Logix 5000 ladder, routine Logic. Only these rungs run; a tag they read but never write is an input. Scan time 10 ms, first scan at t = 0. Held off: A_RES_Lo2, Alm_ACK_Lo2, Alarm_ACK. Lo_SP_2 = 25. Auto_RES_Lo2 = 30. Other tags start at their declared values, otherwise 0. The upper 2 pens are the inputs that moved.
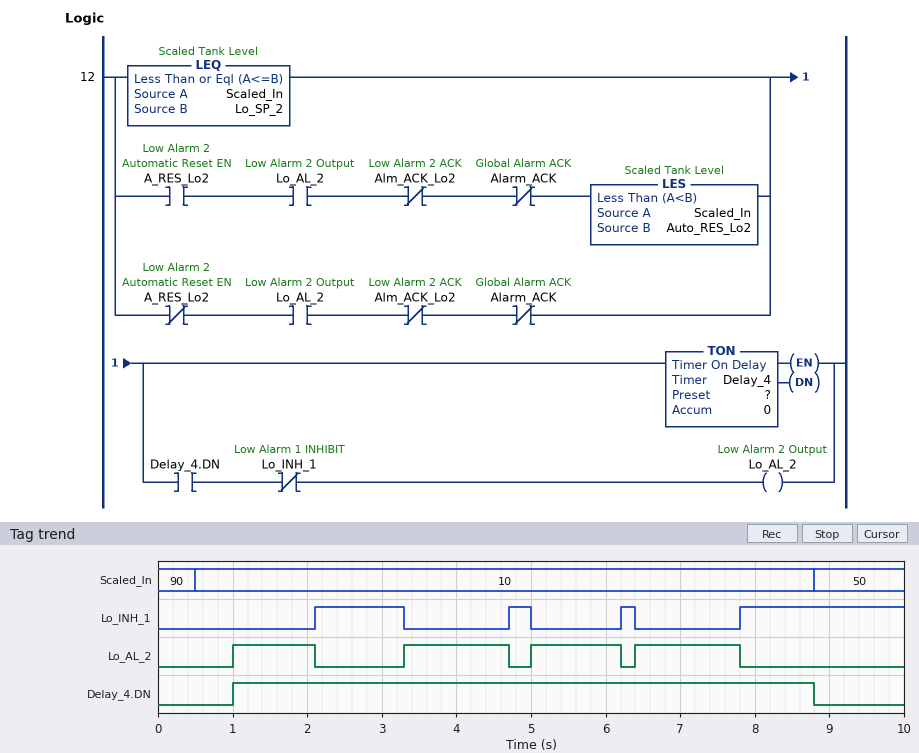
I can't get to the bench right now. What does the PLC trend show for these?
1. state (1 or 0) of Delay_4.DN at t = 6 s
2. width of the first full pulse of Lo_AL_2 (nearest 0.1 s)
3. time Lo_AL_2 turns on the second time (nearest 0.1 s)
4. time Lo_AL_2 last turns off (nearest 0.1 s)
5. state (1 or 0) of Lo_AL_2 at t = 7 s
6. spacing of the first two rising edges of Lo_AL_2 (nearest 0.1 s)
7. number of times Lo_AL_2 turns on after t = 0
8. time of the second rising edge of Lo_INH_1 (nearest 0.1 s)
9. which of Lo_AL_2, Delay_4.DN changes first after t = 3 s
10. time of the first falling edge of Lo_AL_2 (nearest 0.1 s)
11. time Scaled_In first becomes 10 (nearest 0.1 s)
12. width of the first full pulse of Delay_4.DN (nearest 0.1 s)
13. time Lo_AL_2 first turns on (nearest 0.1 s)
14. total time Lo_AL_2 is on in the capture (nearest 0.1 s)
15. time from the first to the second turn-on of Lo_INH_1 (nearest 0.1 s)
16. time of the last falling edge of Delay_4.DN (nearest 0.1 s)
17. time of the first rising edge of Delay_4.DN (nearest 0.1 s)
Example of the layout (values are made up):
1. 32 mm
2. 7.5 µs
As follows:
1. 1
2. 1.1 s
3. 3.3 s
4. 7.8 s
5. 1
6. 2.3 s
7. 4
8. 4.7 s
9. Lo_AL_2
10. 2.1 s
11. 0.5 s
12. 7.8 s
13. 1.0 s
14. 5.1 s
15. 2.6 s
16. 8.8 s
17. 1.0 s
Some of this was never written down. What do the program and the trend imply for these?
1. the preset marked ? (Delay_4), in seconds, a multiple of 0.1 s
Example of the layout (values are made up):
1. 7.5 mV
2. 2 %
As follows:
1. 0.5 s
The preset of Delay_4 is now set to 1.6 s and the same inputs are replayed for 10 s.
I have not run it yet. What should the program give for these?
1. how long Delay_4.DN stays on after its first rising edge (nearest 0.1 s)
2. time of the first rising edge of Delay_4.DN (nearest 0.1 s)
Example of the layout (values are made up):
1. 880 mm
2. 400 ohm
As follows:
1. 6.7 s
2. 2.1 s
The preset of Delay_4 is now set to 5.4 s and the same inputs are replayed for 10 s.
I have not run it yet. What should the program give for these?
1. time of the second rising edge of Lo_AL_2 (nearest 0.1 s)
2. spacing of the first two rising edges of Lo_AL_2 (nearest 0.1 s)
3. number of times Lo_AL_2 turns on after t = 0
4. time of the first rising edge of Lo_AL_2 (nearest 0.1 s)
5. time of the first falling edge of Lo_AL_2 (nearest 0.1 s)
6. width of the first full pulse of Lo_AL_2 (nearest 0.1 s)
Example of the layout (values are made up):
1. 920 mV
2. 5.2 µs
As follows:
1. 6.4 s
2. 0.5 s
3. 2
4. 5.9 s
5. 6.2 s
6. 0.3 s
